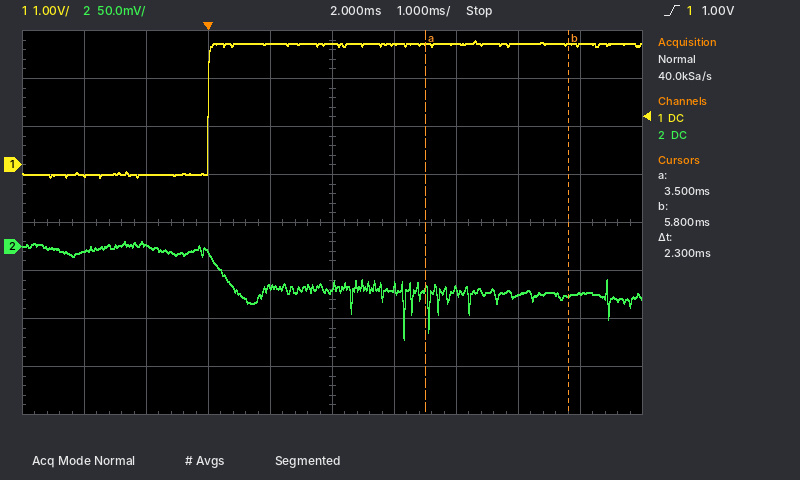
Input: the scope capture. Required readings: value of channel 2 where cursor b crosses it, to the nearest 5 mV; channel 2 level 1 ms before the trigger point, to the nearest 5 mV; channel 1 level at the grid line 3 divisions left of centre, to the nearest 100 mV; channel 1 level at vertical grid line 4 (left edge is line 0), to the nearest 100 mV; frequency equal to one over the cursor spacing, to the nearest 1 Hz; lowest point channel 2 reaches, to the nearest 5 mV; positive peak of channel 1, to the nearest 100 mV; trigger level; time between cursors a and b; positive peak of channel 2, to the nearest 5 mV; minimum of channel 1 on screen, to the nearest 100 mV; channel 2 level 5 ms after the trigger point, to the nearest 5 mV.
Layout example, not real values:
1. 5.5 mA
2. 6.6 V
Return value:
1. -50 mV
2. 0 mV
3. -200 mV
4. 2.5 V
5. 435 Hz
6. -95 mV
7. 2.6 V
8. 1.00 V
9. 2.3 ms
10. 5 mV
11. -300 mV
12. -50 mV
